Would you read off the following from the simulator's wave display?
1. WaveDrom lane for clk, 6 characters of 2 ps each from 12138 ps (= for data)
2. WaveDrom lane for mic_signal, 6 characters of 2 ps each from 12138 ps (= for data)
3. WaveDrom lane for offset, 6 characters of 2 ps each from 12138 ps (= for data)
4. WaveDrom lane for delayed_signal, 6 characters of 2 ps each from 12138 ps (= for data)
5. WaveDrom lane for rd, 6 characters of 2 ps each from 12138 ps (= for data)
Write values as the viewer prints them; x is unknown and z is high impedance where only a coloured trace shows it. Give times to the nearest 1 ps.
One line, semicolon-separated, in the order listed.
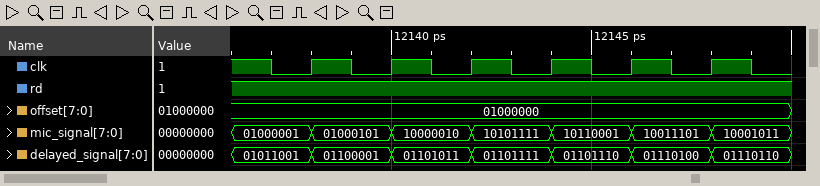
{name: 'clk', wave: 'p.....'}; {name: 'mic_signal', wave: '======', data: '01000101 10000010 10101111 10110001 10011101 10001011'}; {name: 'offset', wave: '=.....', data: '01000000'}; {name: 'delayed_signal', wave: '======', data: '01100001 01101011 01101111 01101110 01110100 01110110'}; {name: 'rd', wave: '1.....'}
